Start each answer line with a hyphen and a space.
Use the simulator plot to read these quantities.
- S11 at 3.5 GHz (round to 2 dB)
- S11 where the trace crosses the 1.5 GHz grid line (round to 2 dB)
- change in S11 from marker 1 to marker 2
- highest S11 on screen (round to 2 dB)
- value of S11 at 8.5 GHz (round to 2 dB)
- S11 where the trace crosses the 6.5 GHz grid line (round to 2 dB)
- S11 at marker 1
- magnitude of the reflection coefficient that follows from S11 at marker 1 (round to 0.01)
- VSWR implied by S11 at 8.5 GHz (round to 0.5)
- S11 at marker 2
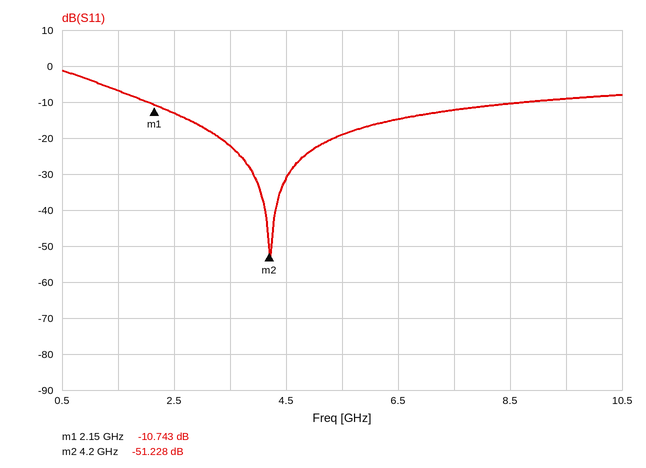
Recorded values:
- -22 dB
- -6 dB
- -40.485 dB
- -2 dB
- -10 dB
- -14 dB
- -10.743 dB
- 0.29
- 2.0
- -51.228 dB
